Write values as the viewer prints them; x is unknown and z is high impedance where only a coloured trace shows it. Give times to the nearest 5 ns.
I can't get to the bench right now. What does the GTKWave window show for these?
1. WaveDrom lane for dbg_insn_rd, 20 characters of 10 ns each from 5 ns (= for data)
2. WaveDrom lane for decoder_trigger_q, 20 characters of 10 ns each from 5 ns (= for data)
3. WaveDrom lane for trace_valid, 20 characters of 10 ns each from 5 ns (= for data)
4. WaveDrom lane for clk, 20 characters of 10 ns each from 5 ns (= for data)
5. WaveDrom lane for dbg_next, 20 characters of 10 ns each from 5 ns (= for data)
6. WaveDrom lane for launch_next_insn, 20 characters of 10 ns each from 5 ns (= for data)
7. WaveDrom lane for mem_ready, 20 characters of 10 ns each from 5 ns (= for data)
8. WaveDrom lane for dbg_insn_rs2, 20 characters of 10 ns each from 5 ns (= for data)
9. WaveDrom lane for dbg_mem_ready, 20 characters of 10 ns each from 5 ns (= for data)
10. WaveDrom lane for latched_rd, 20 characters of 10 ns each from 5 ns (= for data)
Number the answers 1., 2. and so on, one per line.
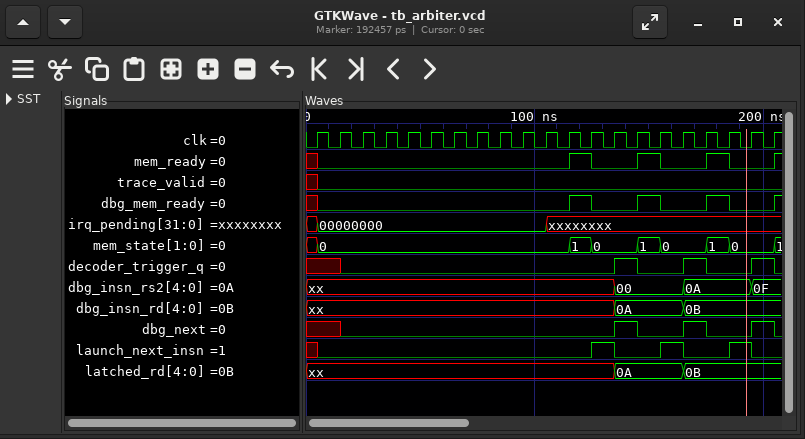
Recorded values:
1. {name: 'dbg_insn_rd', wave: 'x............=..=...', data: '0A 0B'}
2. {name: 'decoder_trigger_q', wave: 'x0...........10.10.1'}
3. {name: 'trace_valid', wave: '0...................'}
4. {name: 'clk', wave: 'p...................'}
5. {name: 'dbg_next', wave: 'x0...........10.10.1'}
6. {name: 'launch_next_insn', wave: '0...........10.10.10'}
7. {name: 'mem_ready', wave: '0..........10.10.10.'}
8. {name: 'dbg_insn_rs2', wave: 'x............=..=..=', data: '00 0A 0F'}
9. {name: 'dbg_mem_ready', wave: '0..........10.10.10.'}
10. {name: 'latched_rd', wave: 'x............=..=...', data: '0A 0B'}
